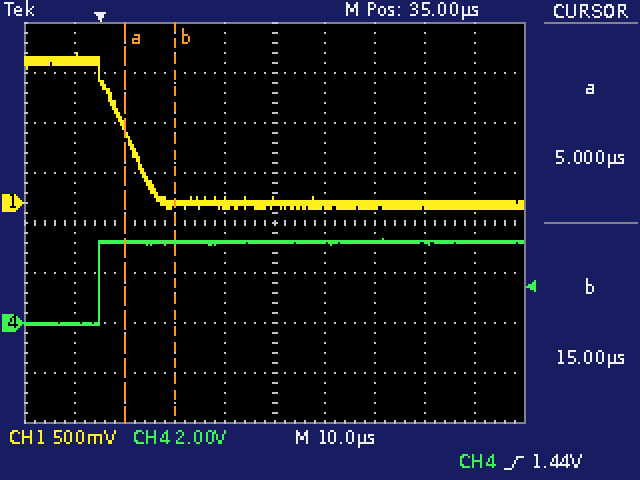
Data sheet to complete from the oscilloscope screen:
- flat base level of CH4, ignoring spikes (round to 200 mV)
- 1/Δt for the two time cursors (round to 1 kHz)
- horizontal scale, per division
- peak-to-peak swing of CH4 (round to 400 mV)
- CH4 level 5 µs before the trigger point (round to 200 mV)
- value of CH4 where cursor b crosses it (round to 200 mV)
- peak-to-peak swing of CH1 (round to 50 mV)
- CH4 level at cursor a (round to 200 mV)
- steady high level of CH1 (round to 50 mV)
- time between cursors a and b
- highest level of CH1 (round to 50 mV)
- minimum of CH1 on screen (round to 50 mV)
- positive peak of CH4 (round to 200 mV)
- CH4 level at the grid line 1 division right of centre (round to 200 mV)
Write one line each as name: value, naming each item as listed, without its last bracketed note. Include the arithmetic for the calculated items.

flat base level of CH4, ignoring spikes: 0.0 V
1/Δt for the two time cursors: 1 / 10 µs ≈ 100 kHz
horizontal scale, per division: 10 µs
peak-to-peak swing of CH4: 3.6 V
CH4 level 5 µs before the trigger point: 0.0 V
value of CH4 where cursor b crosses it: 3.2 V
peak-to-peak swing of CH1: 1.50 V − (-50 mV) = 1.55 V
CH4 level at cursor a: 3.2 V
steady high level of CH1: 1.40 V
time between cursors a and b: 15 µs − (5 µs) = 10 µs
highest level of CH1: 1.50 V
minimum of CH1 on screen: -50 mV
positive peak of CH4: 3.4 V
CH4 level at the grid line 1 division right of centre: 3.2 V
